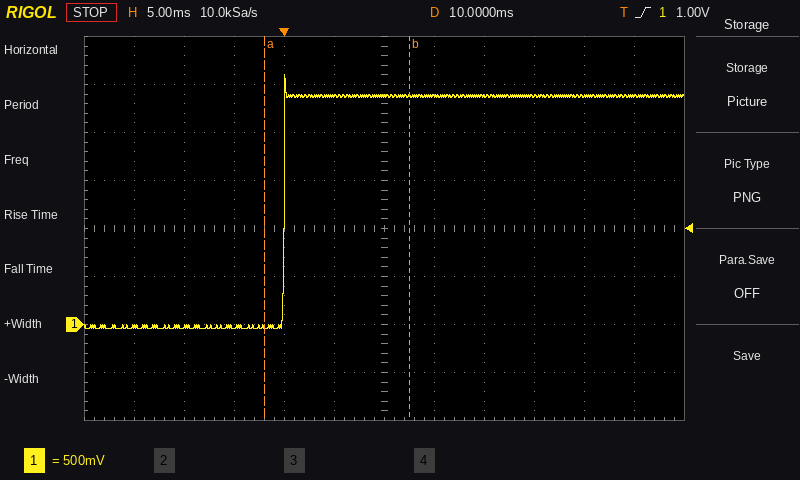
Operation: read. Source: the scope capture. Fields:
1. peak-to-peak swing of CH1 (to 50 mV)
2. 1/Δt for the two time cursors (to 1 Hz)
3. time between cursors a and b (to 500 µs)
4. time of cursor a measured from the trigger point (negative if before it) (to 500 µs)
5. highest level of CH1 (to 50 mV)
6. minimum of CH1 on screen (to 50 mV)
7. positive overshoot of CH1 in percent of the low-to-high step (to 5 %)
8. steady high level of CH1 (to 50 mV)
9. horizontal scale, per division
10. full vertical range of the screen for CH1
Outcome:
2.65 V
69 Hz
14.5 ms
-2.0 ms
2.60 V
-50 mV
10 %
2.40 V
5 ms
4 V
